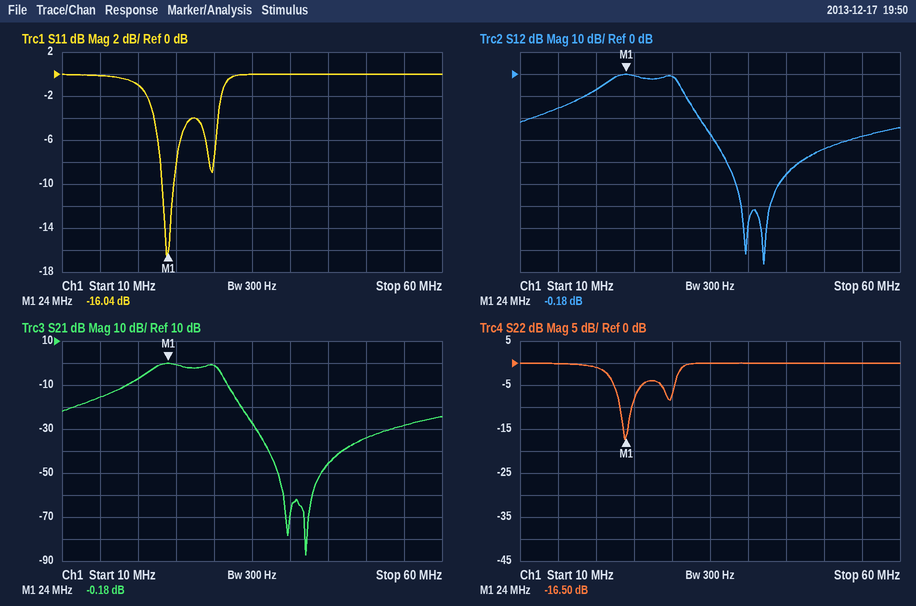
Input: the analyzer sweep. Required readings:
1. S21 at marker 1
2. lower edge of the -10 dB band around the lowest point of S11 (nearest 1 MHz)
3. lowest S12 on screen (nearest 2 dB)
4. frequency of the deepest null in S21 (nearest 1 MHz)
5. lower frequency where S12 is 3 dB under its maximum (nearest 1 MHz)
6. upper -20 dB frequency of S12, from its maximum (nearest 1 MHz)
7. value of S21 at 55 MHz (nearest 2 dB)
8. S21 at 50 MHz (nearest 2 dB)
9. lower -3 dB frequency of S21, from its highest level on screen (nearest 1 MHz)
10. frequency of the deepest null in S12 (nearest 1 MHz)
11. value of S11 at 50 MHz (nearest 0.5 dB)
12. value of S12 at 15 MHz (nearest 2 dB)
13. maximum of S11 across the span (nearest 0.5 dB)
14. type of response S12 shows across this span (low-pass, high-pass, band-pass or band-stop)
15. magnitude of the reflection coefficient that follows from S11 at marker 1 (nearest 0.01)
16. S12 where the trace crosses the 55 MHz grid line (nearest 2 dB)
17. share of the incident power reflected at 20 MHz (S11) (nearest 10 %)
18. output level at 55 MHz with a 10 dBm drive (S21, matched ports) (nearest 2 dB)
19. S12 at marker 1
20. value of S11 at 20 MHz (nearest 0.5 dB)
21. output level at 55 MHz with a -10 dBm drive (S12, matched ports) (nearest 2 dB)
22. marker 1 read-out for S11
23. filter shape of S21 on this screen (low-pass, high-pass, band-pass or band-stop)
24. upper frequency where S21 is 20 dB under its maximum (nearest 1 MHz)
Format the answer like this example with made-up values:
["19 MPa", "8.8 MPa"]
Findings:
["-0.18 dB", "23 MHz", "-86 dB", "42 MHz", "22 MHz", "34 MHz", "-28 dB", "-34 dB", "22 MHz", "42 MHz", "0.0 dB", "-16 dB", "0.0 dB", "band-pass", "0.16", "-28 dB", "80 %", "-18 dBm", "-0.18 dB", "-1.0 dB", "-38 dBm", "-16.04 dB", "band-pass", "34 MHz"]
